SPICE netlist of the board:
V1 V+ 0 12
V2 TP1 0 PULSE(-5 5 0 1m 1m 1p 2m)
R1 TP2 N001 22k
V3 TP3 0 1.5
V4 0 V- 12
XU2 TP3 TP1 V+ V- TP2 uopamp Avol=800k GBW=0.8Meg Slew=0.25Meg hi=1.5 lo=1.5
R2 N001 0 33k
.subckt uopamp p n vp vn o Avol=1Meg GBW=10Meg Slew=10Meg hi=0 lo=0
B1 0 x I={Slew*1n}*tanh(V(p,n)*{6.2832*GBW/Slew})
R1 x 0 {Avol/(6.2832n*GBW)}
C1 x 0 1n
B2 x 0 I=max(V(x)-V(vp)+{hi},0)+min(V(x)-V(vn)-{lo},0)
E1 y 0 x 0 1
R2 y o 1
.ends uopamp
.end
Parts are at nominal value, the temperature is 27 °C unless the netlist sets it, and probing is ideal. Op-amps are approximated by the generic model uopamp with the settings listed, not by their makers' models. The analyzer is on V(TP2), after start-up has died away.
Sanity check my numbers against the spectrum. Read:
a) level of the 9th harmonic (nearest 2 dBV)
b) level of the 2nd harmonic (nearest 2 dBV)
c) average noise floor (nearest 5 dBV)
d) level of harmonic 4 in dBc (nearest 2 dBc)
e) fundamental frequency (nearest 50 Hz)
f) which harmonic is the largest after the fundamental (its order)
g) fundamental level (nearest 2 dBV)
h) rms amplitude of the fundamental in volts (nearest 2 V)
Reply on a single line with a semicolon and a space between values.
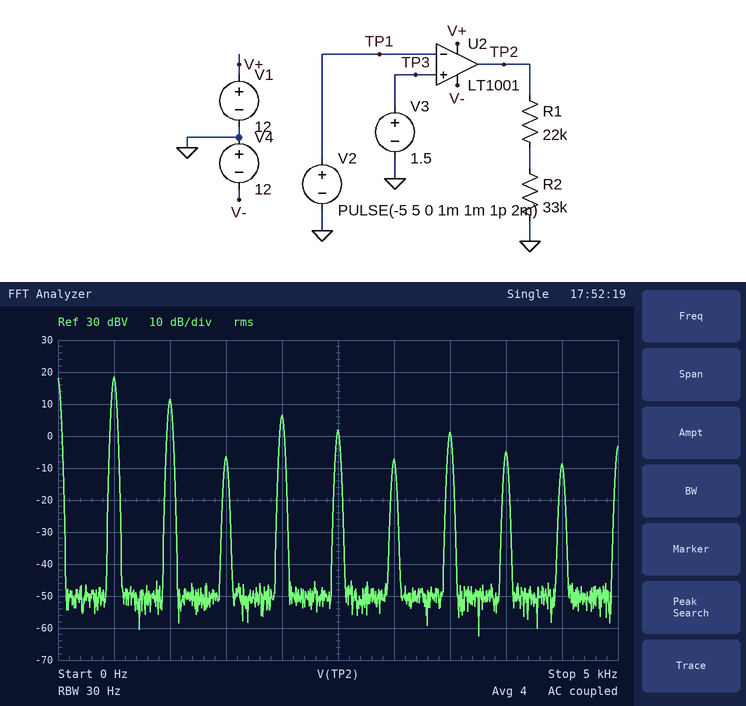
-8 dBV; 12 dBV; -50 dBV; -12 dBc; 500 Hz; 2; 18 dBV; 8 V
